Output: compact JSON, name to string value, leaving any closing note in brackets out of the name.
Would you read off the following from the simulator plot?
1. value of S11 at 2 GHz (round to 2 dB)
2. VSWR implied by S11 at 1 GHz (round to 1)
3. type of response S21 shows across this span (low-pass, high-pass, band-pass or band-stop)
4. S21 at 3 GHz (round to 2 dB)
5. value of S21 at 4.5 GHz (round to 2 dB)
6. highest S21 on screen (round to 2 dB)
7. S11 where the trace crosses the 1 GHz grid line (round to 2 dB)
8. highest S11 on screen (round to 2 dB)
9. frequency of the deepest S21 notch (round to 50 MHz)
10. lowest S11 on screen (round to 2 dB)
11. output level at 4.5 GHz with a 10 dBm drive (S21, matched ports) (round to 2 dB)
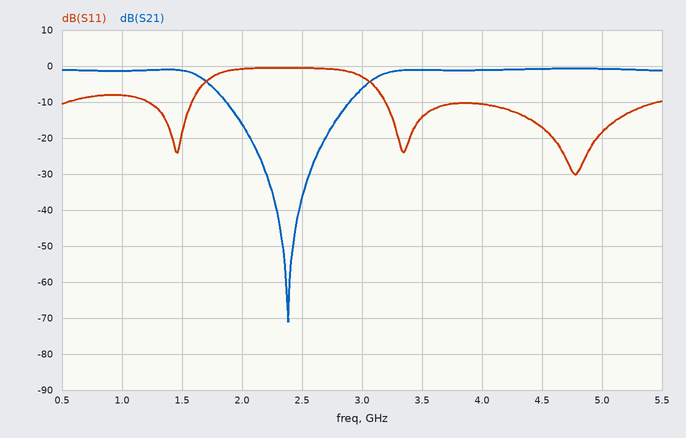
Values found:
{"value of S11 at 2 GHz": "0 dB", "VSWR implied by S11 at 1 GHz": "2", "type of response S21 shows across this span": "band-stop", "S21 at 3 GHz": "-6 dB", "value of S21 at 4.5 GHz": "0 dB", "highest S21 on screen": "0 dB", "S11 where the trace crosses the 1 GHz grid line": "-8 dB", "highest S11 on screen": "0 dB", "frequency of the deepest S21 notch": "2.40 GHz", "lowest S11 on screen": "-30 dB", "output level at 4.5 GHz with a 10 dBm drive (S21, matched ports)": "10 dBm"}
